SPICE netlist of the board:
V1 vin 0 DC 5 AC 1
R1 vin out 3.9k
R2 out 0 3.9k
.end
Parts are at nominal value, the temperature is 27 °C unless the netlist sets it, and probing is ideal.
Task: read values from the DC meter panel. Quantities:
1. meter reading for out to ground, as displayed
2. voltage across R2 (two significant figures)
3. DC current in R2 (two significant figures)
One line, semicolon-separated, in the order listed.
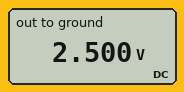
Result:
2.500 V; 2.5 V; 640 µA
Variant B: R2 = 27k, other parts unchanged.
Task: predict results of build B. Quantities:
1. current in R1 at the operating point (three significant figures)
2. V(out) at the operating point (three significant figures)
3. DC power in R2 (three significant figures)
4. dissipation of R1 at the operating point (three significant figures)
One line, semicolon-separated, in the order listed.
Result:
162 µA; 4.37 V; 707 µW; 102 µW
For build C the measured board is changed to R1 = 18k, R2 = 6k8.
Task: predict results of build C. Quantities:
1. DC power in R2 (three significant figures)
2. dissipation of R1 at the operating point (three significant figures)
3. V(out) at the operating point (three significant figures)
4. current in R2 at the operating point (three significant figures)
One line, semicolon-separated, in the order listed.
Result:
276 µW; 732 µW; 1.37 V; 202 µA
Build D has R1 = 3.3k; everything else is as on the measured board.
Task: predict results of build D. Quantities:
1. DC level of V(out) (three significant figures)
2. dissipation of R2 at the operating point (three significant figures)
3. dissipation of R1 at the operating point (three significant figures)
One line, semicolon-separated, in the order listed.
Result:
2.71 V; 1.88 mW; 1.59 mW
